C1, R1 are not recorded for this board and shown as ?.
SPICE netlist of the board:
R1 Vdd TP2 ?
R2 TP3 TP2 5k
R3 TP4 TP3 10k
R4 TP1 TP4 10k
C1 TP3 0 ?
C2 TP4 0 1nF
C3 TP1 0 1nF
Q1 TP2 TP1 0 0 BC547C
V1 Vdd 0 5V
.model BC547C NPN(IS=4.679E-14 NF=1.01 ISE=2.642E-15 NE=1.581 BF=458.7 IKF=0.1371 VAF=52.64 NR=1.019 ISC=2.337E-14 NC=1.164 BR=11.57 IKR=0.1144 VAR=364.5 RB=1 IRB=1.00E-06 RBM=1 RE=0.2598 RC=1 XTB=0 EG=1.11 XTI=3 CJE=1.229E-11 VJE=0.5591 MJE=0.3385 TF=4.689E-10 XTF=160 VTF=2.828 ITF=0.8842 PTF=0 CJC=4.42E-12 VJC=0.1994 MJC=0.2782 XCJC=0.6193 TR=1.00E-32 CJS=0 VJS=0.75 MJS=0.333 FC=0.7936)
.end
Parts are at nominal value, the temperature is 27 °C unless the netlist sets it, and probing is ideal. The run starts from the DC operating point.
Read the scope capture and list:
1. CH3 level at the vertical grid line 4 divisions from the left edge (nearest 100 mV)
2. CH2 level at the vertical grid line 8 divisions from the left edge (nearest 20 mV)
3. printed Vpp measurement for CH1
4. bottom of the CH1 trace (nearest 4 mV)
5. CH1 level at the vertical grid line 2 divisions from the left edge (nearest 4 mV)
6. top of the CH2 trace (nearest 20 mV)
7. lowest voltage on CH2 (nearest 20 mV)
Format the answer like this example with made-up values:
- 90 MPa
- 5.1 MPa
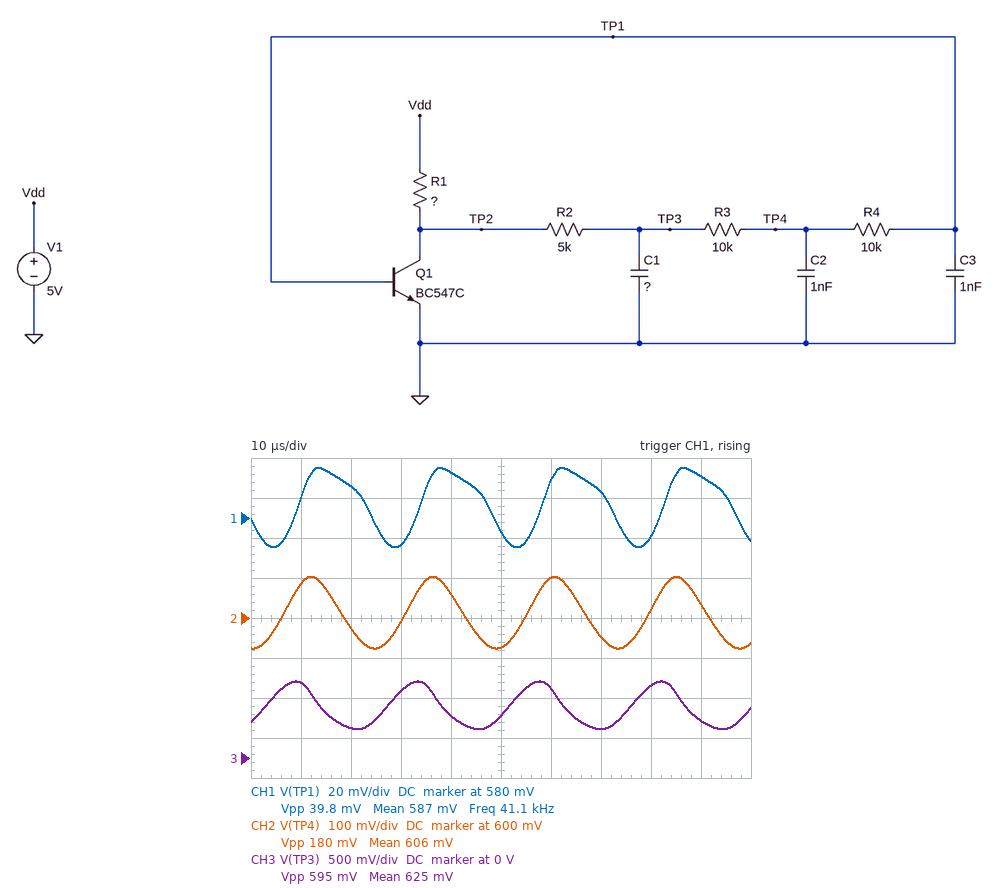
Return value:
- 500 mV
- 620 mV
- 39.8 mV
- 564 mV
- 596 mV
- 700 mV
- 520 mV
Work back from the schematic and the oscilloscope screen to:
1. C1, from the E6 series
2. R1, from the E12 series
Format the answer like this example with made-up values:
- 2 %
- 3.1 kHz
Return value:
- 1.5 nF
- 15 kΩ
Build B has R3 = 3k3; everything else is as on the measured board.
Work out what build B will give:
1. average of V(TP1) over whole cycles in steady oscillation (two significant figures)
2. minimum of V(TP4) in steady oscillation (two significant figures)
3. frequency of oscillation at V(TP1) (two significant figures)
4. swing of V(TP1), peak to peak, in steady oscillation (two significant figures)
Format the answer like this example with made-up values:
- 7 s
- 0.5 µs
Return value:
- 590 mV
- 510 mV
- 59 kHz
- 33 mV
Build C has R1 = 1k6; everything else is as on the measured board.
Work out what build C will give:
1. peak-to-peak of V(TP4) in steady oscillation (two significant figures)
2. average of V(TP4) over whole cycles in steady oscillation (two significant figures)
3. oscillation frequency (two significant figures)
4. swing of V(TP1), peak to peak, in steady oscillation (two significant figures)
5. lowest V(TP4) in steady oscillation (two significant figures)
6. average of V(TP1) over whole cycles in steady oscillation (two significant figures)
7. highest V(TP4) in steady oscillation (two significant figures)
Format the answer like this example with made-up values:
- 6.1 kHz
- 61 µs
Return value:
- 150 mV
- 720 mV
- 55 kHz
- 18 mV
- 640 mV
- 650 mV
- 790 mV
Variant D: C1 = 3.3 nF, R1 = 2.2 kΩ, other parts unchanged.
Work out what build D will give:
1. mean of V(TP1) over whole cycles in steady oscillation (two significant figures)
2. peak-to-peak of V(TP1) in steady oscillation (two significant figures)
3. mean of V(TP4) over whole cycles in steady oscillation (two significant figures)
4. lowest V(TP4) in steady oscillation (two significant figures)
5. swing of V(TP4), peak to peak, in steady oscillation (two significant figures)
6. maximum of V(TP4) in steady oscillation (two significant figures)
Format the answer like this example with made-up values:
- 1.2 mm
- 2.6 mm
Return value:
- 640 mV
- 18 mV
- 690 mV
- 630 mV
- 120 mV
- 750 mV
